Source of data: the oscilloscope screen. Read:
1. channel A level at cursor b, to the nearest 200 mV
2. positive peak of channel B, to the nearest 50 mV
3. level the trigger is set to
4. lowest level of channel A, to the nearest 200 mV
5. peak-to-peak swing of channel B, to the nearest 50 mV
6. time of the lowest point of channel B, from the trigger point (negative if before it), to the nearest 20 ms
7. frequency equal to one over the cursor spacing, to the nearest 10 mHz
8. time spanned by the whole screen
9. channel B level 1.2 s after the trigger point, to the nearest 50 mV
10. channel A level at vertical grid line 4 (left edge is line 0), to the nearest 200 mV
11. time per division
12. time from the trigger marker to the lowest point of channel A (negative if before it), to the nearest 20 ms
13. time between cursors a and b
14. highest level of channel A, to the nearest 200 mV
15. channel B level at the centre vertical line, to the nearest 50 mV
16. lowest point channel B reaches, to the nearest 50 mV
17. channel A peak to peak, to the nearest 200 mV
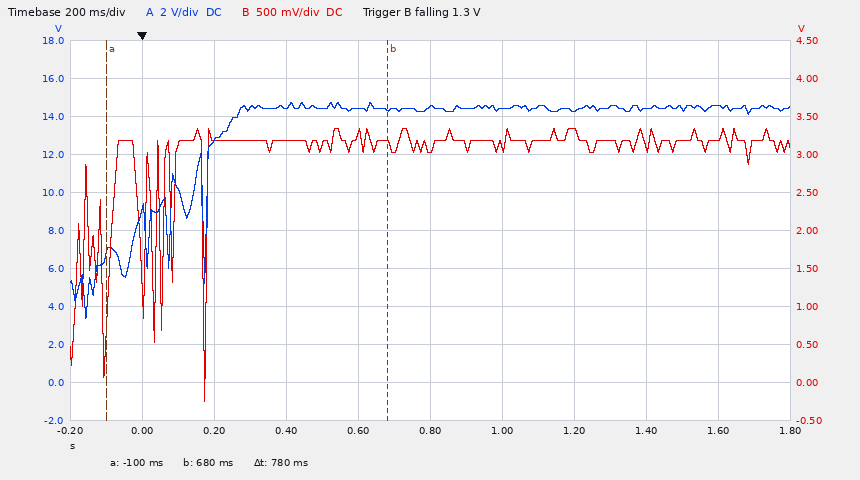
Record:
14.4 V
3.35 V
1.3 V
3.4 V
3.60 V
+180 ms
1.28 Hz
2 s
3.30 V
14.4 V
200 ms
-160 ms
780 ms
14.8 V
3.05 V
-250 mV
11.4 V
